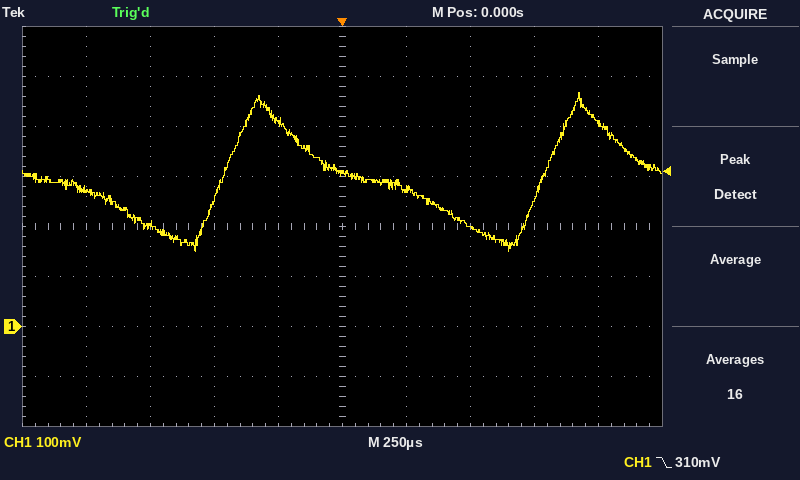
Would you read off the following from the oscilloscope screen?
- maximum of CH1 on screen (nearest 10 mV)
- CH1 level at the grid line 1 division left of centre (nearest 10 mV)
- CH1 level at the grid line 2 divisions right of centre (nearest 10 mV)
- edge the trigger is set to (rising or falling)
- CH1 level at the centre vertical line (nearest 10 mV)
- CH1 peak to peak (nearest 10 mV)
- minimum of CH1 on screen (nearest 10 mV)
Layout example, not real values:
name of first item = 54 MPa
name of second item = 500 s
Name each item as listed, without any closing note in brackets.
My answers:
maximum of CH1 on screen = 470 mV
CH1 level at the grid line 1 division left of centre = 410 mV
CH1 level at the grid line 2 divisions right of centre = 200 mV
edge the trigger is set to = falling
CH1 level at the centre vertical line = 310 mV
CH1 peak to peak = 320 mV
minimum of CH1 on screen = 150 mV
